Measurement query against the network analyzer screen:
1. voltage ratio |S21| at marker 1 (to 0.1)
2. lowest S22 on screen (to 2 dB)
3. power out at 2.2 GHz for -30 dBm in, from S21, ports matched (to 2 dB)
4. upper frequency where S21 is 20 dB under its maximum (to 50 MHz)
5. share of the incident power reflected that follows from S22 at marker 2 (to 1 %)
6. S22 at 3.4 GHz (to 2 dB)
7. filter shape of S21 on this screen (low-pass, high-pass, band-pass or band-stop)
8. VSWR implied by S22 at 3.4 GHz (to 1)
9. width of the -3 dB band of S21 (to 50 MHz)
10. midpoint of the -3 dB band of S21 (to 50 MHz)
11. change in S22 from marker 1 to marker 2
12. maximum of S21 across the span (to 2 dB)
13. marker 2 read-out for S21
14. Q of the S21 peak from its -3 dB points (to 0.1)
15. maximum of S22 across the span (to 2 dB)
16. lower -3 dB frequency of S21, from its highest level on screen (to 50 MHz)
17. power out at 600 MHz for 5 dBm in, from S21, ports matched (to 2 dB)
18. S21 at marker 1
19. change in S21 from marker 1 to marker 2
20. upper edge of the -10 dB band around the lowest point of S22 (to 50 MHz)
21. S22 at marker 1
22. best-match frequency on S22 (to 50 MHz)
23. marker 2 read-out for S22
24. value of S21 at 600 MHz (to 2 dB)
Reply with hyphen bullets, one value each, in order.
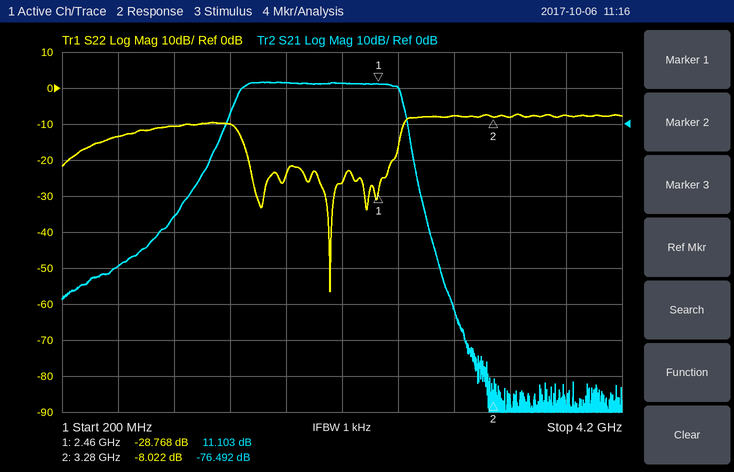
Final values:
- 3.6
- -56 dB
- -18 dBm
- 2.70 GHz
- 16 %
- -8 dB
- band-pass
- 2
- 1.15 GHz
- 2.05 GHz
- 20.746 dB
- 12 dB
- -76.492 dB
- 1.8
- -8 dB
- 1.45 GHz
- -34 dBm
- 11.103 dB
- -87.595 dB
- 2.65 GHz
- -28.768 dB
- 2.10 GHz
- -8.022 dB
- -40 dB
